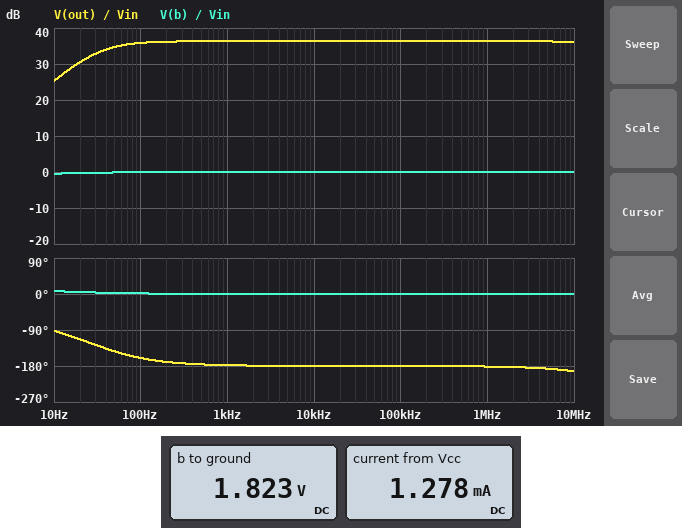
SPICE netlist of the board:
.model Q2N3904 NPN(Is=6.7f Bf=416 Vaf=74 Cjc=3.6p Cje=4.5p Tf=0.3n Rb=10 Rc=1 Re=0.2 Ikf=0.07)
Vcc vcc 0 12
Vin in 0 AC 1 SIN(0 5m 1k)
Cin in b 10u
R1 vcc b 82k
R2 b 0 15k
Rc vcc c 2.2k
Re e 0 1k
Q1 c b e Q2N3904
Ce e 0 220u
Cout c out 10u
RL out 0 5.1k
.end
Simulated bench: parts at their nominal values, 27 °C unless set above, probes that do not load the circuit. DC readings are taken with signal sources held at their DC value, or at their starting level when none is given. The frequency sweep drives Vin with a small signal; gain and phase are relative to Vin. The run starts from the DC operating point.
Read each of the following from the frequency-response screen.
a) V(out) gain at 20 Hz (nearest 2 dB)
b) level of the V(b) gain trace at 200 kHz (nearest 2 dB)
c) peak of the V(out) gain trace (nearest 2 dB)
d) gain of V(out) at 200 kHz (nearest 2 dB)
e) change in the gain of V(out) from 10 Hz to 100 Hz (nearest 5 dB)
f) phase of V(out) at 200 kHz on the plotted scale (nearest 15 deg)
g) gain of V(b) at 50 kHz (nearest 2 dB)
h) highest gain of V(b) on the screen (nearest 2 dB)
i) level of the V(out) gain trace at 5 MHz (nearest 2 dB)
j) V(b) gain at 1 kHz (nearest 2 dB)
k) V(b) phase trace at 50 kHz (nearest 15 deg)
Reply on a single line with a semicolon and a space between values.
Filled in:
30 dB; 0 dB; 36 dB; 36 dB; 10 dB; -180 deg; 0 dB; 0 dB; 36 dB; 0 dB; 0 deg
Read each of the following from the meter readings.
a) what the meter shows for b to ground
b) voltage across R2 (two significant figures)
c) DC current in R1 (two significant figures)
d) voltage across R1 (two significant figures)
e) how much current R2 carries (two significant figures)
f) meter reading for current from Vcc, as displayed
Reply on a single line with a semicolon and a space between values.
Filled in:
1.823 V; 1.8 V; 120 µA; 10 V; 120 µA; 1.278 mA
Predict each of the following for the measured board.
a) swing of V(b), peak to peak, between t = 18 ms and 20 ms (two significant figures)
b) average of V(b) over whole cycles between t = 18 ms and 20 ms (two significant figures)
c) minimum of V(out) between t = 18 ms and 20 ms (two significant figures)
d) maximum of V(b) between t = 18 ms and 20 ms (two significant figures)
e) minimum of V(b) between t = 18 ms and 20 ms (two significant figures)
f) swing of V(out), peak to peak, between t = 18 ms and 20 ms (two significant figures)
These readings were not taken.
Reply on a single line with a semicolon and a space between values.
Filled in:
10 mV; 1.8 V; -340 mV; 1.8 V; 1.8 V; 650 mV
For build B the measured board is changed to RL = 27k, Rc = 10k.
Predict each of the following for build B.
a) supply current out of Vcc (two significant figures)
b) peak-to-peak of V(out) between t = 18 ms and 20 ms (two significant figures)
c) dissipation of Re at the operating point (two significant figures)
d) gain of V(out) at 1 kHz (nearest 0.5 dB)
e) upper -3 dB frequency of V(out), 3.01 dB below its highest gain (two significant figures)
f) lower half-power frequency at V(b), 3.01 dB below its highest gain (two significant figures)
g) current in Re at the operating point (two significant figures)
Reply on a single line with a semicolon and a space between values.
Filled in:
1.2 mA; 1.8 V; 1.2 mW; 36.0 dB; 14 MHz; 230 Hz; 1.1 mA
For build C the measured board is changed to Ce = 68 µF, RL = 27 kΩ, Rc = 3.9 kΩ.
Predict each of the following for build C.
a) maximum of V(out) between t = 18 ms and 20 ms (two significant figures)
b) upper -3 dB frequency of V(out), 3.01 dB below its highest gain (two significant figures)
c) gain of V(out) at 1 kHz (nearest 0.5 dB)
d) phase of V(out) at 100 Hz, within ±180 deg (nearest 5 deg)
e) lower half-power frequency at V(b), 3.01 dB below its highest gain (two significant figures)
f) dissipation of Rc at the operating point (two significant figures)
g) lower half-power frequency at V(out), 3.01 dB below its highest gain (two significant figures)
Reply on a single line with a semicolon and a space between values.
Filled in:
670 mV; 19 MHz; 43.0 dB; -135 deg; 1.3 Hz; 5.2 mW; 100 Hz
